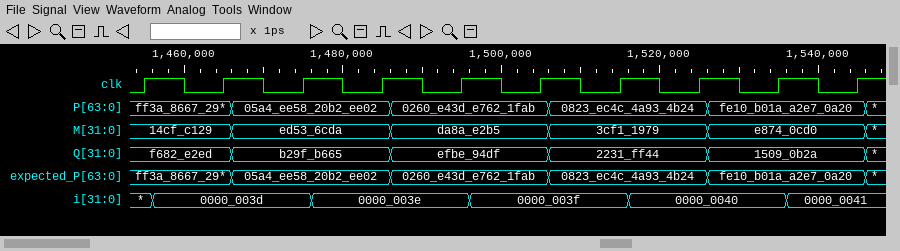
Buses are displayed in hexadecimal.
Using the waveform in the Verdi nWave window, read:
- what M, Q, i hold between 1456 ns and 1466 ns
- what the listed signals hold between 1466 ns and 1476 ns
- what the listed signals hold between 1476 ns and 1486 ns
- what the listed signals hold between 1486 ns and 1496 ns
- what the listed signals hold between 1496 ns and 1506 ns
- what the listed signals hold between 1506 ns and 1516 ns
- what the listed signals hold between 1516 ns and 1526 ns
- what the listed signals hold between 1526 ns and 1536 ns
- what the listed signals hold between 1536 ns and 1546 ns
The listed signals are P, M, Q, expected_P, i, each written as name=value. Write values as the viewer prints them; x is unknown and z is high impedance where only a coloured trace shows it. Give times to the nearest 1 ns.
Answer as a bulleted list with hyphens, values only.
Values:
- M=14cf_c129, Q=f682_e2ed, i=0000_003d
- P=05a4_ee58_20b2_ee02, M=ed53_6cda, Q=b29f_b665, expected_P=05a4_ee58_20b2_ee02, i=0000_003d
- P=05a4_ee58_20b2_ee02, M=ed53_6cda, Q=b29f_b665, expected_P=05a4_ee58_20b2_ee02, i=0000_003e
- P=0260_e43d_e762_1fab, M=da8a_e2b5, Q=efbe_94df, expected_P=0260_e43d_e762_1fab, i=0000_003e
- P=0260_e43d_e762_1fab, M=da8a_e2b5, Q=efbe_94df, expected_P=0260_e43d_e762_1fab, i=0000_003f
- P=0823_ec4c_4a93_4b24, M=3cf1_1979, Q=2231_ff44, expected_P=0823_ec4c_4a93_4b24, i=0000_003f
- P=0823_ec4c_4a93_4b24, M=3cf1_1979, Q=2231_ff44, expected_P=0823_ec4c_4a93_4b24, i=0000_0040
- P=fe10_b01a_a2e7_0a20, M=e874_0cd0, Q=1509_0b2a, expected_P=fe10_b01a_a2e7_0a20, i=0000_0040
- P=fe10_b01a_a2e7_0a20, M=e874_0cd0, Q=1509_0b2a, expected_P=fe10_b01a_a2e7_0a20, i=0000_0041
